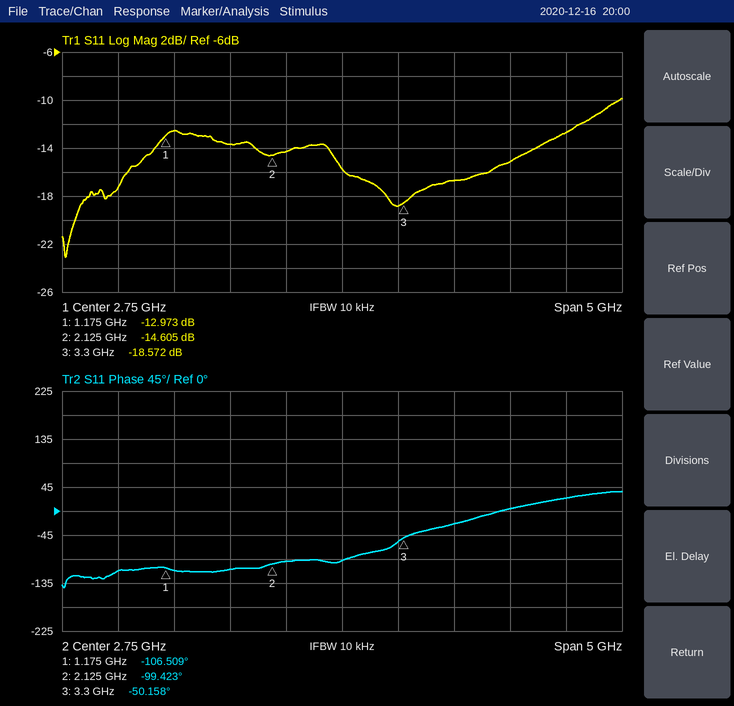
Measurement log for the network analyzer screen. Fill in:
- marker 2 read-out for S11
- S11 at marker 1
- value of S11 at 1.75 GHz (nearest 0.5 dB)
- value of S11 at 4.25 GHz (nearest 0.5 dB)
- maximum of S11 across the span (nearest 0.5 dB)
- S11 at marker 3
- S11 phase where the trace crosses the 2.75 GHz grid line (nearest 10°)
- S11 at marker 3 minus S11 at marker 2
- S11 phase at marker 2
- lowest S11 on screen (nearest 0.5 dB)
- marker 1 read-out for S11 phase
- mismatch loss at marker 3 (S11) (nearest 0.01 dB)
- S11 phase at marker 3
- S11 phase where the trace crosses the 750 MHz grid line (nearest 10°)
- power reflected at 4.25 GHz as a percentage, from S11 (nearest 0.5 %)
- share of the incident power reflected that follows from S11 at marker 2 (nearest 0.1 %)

-14.605 dB
-12.973 dB
-13.5 dB
-15.0 dB
-10.0 dB
-18.572 dB
-90°
-3.967 dB
-99.423°
-23.0 dB
-106.509°
0.06 dB
-50.158°
-110°
3.0 %
3.5 %
